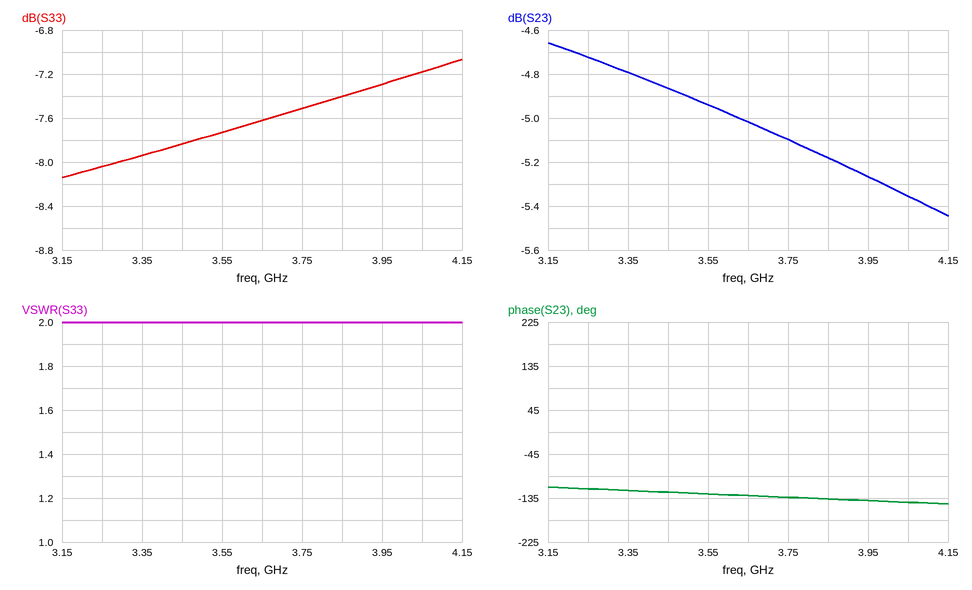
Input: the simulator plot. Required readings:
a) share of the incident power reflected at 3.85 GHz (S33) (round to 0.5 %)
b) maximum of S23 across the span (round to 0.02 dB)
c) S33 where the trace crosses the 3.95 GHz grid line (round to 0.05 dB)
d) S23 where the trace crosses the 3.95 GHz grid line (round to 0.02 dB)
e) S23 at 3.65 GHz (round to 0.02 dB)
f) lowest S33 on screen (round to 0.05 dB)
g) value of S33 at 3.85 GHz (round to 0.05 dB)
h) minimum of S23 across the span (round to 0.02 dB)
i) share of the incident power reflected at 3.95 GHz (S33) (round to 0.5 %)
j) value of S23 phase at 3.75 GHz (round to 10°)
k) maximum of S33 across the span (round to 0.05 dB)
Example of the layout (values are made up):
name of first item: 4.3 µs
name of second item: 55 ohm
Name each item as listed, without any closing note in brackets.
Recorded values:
share of the incident power reflected at 3.85 GHz (S33): 18.0 %
maximum of S23 across the span: -4.66 dB
S33 where the trace crosses the 3.95 GHz grid line: -7.30 dB
S23 where the trace crosses the 3.95 GHz grid line: -5.26 dB
S23 at 3.65 GHz: -5.02 dB
lowest S33 on screen: -8.15 dB
value of S33 at 3.85 GHz: -7.40 dB
minimum of S23 across the span: -5.44 dB
share of the incident power reflected at 3.95 GHz (S33): 18.5 %
value of S23 phase at 3.75 GHz: -130°
maximum of S33 across the span: -7.05 dB
